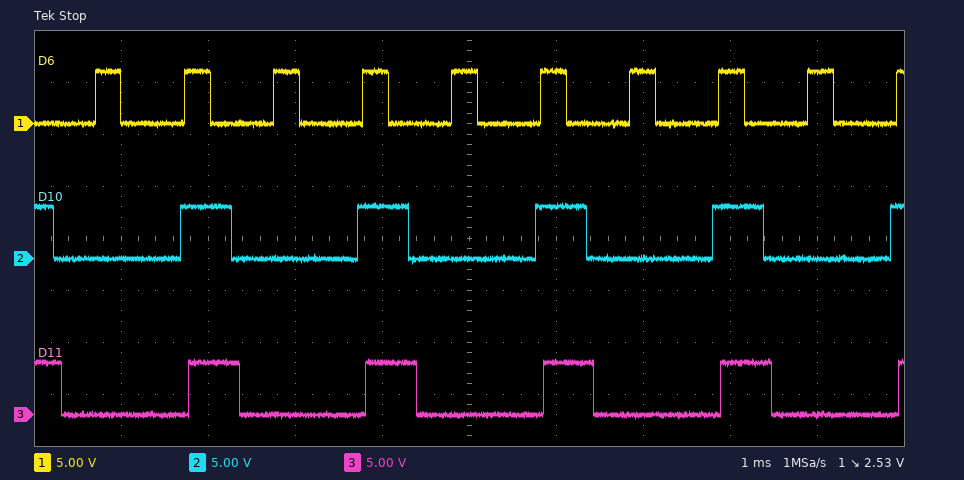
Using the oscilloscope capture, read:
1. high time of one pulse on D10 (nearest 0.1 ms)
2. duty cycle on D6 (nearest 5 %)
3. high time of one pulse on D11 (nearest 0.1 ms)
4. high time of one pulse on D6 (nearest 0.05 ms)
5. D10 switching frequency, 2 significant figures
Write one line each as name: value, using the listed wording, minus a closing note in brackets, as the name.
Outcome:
high time of one pulse on D10: 0.6 ms
duty cycle on D6: 30 %
high time of one pulse on D11: 0.6 ms
high time of one pulse on D6: 0.30 ms
D10 switching frequency, 2 significant figures: 490 Hz
